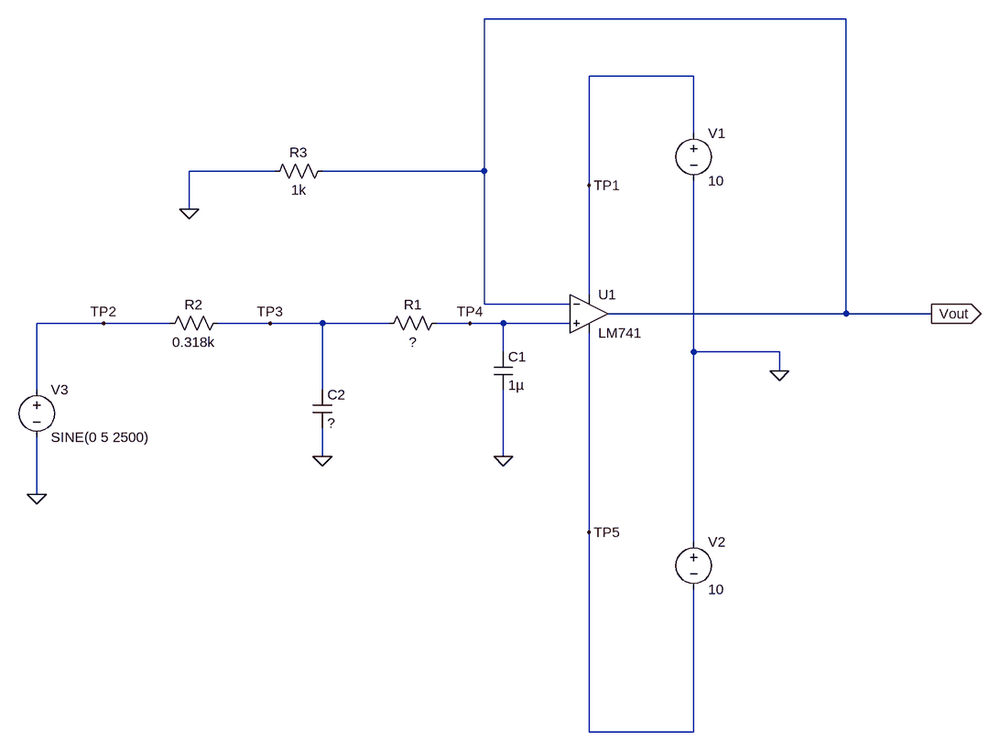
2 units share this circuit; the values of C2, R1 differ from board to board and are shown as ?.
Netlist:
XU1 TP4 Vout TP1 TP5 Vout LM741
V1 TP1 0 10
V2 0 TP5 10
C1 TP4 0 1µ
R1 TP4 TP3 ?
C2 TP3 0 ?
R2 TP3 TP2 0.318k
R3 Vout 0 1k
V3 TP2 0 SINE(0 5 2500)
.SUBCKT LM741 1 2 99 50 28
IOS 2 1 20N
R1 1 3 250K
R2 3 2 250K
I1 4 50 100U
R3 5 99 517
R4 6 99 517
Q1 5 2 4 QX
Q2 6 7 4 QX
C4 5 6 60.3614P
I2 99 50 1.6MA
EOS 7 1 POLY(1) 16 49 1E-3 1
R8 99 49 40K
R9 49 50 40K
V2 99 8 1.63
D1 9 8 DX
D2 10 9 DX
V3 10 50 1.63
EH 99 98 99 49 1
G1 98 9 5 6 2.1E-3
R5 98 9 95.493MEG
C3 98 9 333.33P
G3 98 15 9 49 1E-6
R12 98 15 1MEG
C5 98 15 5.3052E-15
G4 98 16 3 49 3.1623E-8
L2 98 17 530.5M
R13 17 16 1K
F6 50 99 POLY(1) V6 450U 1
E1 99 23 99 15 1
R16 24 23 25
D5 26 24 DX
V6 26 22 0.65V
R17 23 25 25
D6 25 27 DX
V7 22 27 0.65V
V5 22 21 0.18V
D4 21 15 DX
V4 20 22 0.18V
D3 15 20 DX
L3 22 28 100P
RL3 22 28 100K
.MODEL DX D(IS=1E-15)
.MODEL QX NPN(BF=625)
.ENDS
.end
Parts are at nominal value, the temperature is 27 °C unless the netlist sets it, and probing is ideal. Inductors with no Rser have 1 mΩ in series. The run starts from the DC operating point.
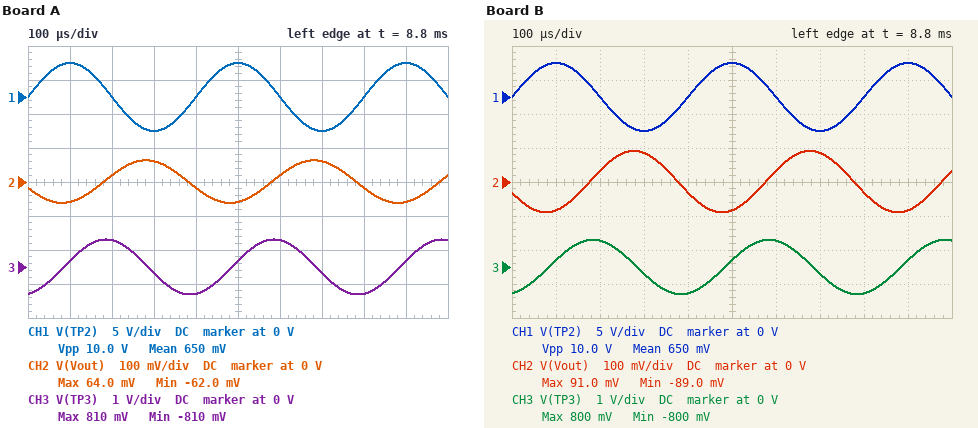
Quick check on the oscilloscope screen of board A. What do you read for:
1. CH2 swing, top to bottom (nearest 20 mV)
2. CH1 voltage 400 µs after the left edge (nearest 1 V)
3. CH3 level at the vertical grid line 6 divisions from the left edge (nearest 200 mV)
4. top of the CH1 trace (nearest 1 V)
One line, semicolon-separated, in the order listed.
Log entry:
120 mV; 0 V; 800 mV; 5 V
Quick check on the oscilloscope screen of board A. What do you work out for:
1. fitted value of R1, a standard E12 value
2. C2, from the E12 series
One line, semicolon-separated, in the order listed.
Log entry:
820 Ω; 1.2 µF
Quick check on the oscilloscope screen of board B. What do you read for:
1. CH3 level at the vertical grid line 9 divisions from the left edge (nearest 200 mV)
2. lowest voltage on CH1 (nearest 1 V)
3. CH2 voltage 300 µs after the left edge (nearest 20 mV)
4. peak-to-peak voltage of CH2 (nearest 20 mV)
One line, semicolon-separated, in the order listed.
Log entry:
200 mV; -5 V; 80 mV; 180 mV
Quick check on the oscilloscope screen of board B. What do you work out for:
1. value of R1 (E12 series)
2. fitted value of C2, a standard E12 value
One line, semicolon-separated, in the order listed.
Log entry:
560 Ω; 1.2 µF
